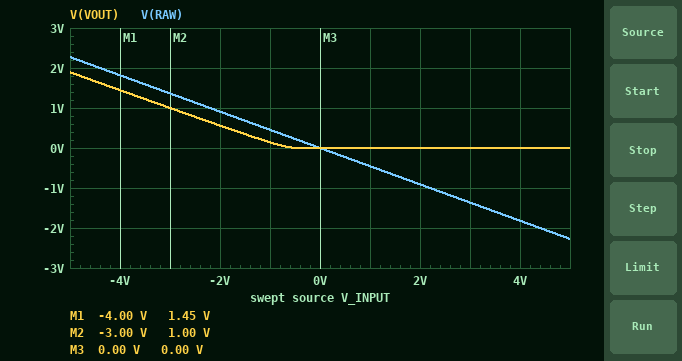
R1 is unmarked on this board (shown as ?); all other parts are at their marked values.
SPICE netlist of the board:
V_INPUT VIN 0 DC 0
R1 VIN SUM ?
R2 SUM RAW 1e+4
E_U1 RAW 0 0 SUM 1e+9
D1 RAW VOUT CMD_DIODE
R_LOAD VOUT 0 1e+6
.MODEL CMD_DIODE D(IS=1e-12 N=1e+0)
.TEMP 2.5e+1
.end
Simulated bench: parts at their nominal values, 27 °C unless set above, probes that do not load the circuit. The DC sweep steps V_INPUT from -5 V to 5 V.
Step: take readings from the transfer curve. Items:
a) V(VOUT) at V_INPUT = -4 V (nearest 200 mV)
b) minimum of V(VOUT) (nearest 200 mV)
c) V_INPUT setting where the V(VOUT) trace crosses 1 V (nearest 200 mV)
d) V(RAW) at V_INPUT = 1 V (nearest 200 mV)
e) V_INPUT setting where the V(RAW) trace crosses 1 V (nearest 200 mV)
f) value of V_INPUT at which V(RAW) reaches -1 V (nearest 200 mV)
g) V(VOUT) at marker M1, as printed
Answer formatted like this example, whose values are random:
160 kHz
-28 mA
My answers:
1.4 V
0 V
-3.0 V
-400 mV
-2.2 V
2.2 V
1.45 V
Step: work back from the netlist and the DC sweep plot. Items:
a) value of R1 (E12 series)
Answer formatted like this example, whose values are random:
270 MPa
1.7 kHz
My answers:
22 kΩ
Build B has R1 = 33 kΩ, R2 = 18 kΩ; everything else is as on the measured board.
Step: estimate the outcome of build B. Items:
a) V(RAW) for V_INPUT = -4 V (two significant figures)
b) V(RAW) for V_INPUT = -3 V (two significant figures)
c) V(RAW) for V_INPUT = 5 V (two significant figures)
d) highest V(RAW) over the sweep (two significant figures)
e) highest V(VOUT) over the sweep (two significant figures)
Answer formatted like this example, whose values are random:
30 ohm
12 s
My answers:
2.2 V
1.6 V
-2.7 V
2.7 V
2.3 V
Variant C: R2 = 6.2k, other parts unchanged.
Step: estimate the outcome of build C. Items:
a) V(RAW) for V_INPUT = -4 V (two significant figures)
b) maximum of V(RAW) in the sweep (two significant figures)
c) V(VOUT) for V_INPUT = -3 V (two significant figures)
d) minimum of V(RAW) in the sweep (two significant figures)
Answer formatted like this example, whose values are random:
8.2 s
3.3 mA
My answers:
1.1 V
1.4 V
500 mV
-1.4 V
